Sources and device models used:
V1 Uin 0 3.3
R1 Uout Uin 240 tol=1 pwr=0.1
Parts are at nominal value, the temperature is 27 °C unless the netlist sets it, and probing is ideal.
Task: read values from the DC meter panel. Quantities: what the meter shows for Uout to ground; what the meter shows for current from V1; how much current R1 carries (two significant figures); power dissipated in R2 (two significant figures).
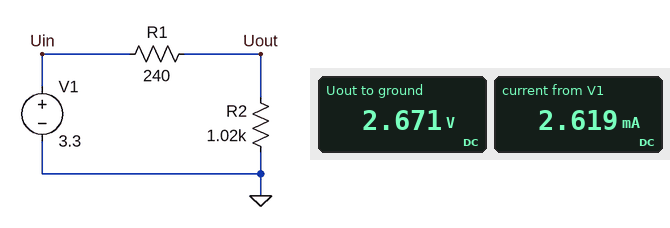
2.671 V
2.619 mA
2.6 mA
7.0 mW
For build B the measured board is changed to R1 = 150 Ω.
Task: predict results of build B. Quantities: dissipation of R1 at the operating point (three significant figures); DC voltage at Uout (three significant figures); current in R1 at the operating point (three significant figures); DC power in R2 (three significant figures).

1.19 mW
2.88 V
2.82 mA
8.11 mW
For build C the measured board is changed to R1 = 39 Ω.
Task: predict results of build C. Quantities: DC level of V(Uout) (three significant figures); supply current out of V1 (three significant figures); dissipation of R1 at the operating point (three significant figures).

3.18 V
3.12 mA
379 µW
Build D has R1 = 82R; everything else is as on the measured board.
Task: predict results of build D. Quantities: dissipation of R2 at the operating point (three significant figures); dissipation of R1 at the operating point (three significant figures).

9.15 mW
735 µW
